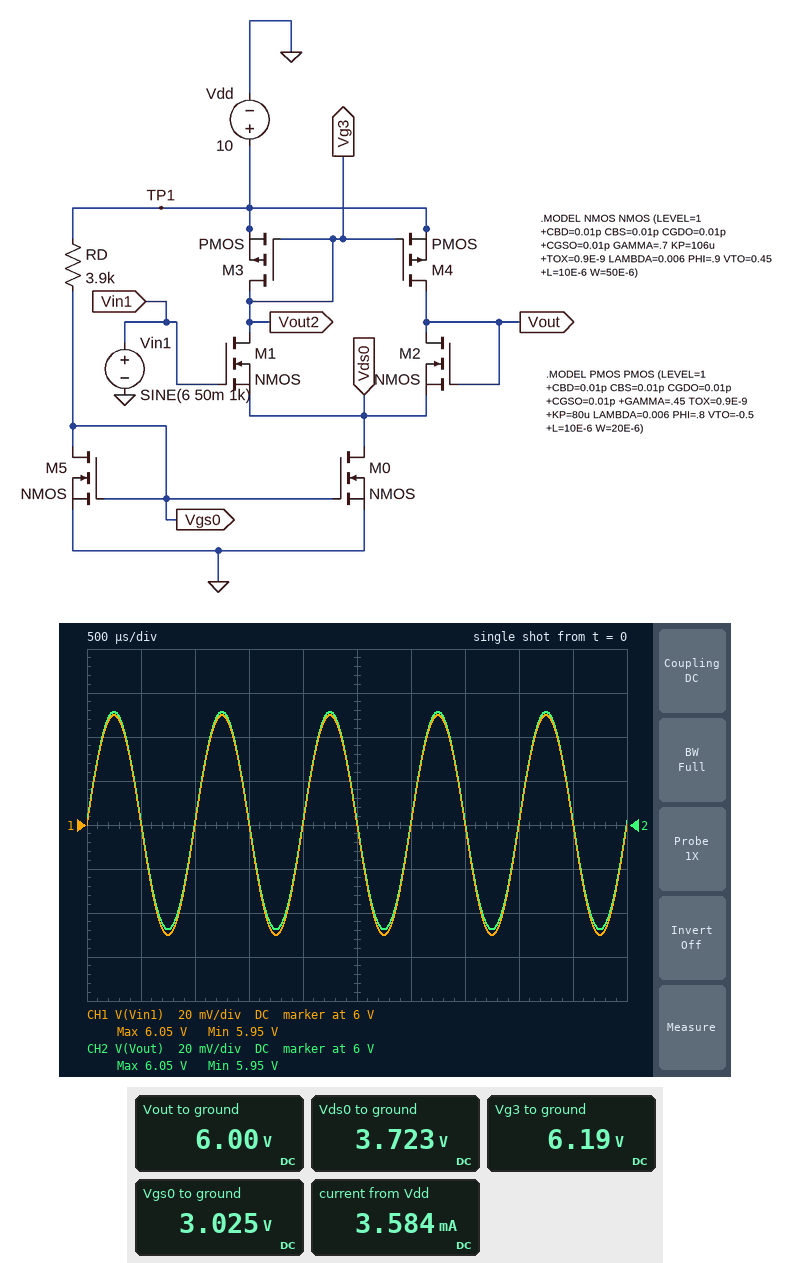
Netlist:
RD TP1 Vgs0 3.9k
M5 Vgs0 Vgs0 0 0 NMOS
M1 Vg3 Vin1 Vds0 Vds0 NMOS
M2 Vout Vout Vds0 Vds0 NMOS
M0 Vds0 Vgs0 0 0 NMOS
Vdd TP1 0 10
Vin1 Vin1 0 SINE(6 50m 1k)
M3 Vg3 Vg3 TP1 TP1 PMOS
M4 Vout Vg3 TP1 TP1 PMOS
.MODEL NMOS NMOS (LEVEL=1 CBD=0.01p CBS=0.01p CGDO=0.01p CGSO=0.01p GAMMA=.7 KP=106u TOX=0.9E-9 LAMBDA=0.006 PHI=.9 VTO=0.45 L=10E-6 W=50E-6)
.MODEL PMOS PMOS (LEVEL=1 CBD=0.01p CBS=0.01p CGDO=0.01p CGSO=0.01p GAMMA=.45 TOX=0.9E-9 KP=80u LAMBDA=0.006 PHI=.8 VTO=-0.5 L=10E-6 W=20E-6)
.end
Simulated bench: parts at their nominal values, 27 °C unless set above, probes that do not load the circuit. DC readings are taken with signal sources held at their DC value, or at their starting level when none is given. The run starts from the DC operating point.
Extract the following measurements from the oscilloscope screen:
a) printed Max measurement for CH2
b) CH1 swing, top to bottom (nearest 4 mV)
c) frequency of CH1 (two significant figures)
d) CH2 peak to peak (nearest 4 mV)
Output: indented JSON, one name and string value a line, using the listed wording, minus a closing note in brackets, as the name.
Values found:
{
  "printed Max measurement for CH2": "6.05 V",
  "CH1 swing, top to bottom": "100 mV",
  "frequency of CH1": "1.0 kHz",
  "CH2 peak to peak": "100 mV"
}
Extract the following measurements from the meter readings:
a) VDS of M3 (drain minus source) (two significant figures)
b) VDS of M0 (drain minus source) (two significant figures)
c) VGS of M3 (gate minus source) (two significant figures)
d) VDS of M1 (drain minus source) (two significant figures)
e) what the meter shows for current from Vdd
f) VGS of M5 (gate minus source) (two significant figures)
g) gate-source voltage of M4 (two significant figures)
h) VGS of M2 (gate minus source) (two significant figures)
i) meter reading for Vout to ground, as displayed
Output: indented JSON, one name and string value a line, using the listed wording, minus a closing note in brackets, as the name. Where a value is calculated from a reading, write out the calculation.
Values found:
{
  "VDS of M3 (drain minus source)": "6.19 V - 10 V = -3.8 V",
  "VDS of M0 (drain minus source)": "3.723 V = 3.7 V",
  "VGS of M3 (gate minus source)": "6.19 V - 10 V = -3.8 V",
  "VDS of M1 (drain minus source)": "6.19 V - 3.723 V = 2.5 V",
  "what the meter shows for current from Vdd": "3.584 mA",
  "VGS of M5 (gate minus source)": "3.025 V = 3.0 V",
  "gate-source voltage of M4": "6.19 V - 10 V = -3.8 V",
  "VGS of M2 (gate minus source)": "6 V - 3.723 V = 2.3 V",
  "meter reading for Vout to ground, as displayed": "6.00 V"
}
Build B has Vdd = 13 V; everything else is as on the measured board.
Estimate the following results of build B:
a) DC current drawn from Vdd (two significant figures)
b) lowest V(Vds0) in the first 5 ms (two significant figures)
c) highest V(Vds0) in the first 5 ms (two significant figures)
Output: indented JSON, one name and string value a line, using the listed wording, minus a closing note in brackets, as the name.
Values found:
{
  "DC current drawn from Vdd": "4.9 mA",
  "lowest V(Vds0) in the first 5 ms": "3.4 V",
  "highest V(Vds0) in the first 5 ms": "3.5 V"
}
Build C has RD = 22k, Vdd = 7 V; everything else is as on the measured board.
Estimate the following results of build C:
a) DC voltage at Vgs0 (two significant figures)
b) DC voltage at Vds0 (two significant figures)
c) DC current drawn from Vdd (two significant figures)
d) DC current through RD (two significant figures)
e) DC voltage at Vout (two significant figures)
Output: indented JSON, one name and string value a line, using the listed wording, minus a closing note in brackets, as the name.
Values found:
{
  "DC voltage at Vgs0": "1.4 V",
  "DC voltage at Vds0": "4.8 V",
  "DC current drawn from Vdd": "510 µA",
  "DC current through RD": "250 µA",
  "DC voltage at Vout": "5.9 V"
}
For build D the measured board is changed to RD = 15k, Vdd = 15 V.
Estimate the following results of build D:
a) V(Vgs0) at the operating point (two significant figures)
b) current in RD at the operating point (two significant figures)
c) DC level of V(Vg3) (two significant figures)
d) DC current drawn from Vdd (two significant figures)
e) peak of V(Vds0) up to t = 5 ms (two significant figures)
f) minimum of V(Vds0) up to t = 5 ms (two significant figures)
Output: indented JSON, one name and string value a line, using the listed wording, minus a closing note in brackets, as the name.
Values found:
{
  "V(Vgs0) at the operating point": "2.2 V",
  "current in RD at the operating point": "850 µA",
  "DC level of V(Vg3)": "12 V",
  "DC current drawn from Vdd": "1.7 mA",
  "peak of V(Vds0) up to t = 5 ms": "4.4 V",
  "minimum of V(Vds0) up to t = 5 ms": "4.3 V"
}
